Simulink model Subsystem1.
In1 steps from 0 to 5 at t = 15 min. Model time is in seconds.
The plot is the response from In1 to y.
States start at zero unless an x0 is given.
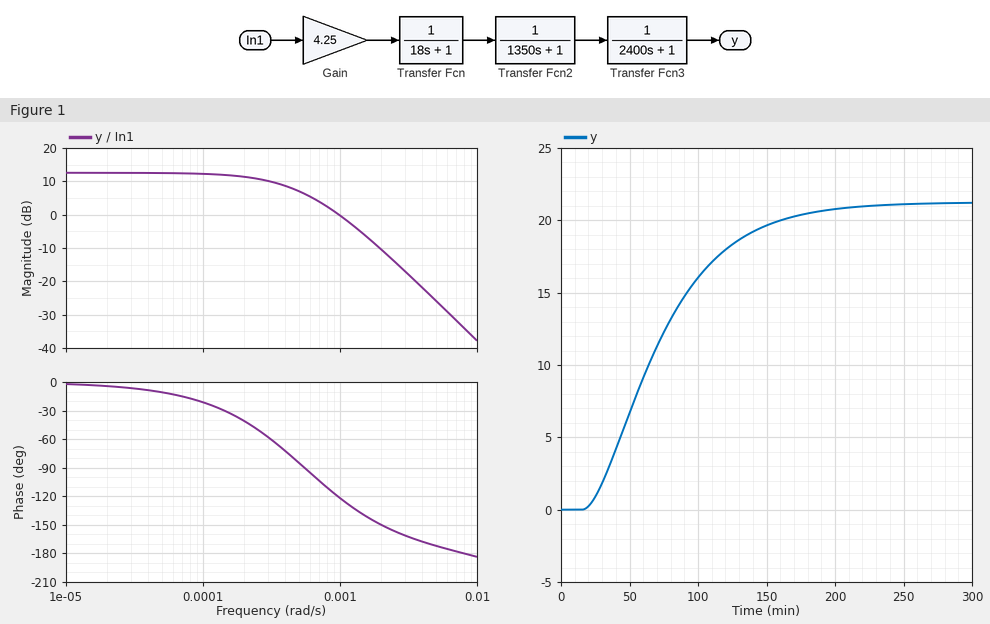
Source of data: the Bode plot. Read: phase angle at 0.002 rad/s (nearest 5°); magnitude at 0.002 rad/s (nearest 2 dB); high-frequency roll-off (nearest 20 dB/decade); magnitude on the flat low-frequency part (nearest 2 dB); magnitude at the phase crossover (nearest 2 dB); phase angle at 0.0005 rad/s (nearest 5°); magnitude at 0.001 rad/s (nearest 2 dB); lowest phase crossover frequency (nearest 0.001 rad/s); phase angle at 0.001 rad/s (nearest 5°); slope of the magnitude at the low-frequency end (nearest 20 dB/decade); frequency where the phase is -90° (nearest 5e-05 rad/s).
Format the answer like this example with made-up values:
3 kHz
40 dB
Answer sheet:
-150°
-10 dB
-40 dB/decade
12 dB
-34 dB
-85°
0 dB
0.008 rad/s
-120°
0 dB/decade
0.00055 rad/s
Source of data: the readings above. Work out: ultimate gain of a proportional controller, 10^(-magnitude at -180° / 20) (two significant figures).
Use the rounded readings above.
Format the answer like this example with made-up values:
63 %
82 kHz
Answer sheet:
50
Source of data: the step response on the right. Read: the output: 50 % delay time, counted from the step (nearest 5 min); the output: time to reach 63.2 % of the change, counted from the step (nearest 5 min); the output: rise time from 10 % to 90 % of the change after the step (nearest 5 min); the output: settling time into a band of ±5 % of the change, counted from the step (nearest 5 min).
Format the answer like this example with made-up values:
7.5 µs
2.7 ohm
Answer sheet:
50 min
65 min
105 min
150 min
